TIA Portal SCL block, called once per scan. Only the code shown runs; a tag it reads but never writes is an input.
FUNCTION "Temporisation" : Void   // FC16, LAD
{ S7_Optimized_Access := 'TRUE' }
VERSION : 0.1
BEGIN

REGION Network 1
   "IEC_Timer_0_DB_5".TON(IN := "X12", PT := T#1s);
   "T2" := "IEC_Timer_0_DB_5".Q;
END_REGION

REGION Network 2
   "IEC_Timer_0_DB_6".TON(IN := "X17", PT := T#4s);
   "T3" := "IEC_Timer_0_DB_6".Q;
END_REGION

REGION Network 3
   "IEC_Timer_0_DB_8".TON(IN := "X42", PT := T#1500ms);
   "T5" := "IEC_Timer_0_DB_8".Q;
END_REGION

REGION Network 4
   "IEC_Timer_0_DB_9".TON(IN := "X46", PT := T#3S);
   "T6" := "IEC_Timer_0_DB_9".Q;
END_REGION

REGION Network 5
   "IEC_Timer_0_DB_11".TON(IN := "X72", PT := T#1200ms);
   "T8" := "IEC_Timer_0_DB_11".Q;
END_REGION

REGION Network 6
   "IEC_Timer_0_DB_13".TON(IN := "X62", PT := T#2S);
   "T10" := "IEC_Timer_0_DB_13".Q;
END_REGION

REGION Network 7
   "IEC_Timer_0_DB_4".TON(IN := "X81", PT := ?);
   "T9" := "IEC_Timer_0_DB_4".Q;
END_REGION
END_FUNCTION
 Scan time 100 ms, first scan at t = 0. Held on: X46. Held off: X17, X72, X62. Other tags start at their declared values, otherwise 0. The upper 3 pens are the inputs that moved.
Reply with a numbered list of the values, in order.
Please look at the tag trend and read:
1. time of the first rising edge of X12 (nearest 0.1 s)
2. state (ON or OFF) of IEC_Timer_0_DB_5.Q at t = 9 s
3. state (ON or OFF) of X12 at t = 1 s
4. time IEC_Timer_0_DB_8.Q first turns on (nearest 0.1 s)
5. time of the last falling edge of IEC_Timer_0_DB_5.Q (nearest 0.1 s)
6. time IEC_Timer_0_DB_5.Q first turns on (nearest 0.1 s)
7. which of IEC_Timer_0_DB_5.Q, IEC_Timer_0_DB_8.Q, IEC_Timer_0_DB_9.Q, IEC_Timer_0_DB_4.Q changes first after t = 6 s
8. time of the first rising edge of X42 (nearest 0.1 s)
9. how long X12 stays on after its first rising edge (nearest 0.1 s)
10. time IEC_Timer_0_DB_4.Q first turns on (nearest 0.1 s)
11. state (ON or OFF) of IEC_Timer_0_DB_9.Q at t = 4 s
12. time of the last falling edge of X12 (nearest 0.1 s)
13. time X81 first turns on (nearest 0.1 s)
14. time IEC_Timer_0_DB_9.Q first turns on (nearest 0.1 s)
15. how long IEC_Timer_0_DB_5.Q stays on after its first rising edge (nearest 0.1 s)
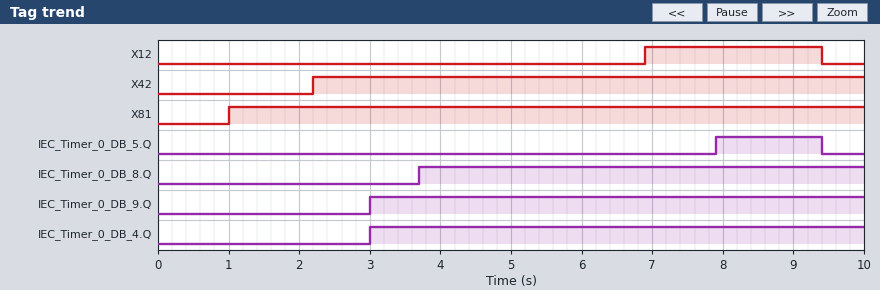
1. 6.9 s
2. ON
3. OFF
4. 3.7 s
5. 9.4 s
6. 7.9 s
7. IEC_Timer_0_DB_5.Q
8. 2.2 s
9. 2.5 s
10. 3.0 s
11. ON
12. 9.4 s
13. 1.0 s
14. 3.0 s
15. 1.5 s
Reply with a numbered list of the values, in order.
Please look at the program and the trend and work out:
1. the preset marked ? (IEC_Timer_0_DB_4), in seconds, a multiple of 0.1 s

1. 2.0 s
